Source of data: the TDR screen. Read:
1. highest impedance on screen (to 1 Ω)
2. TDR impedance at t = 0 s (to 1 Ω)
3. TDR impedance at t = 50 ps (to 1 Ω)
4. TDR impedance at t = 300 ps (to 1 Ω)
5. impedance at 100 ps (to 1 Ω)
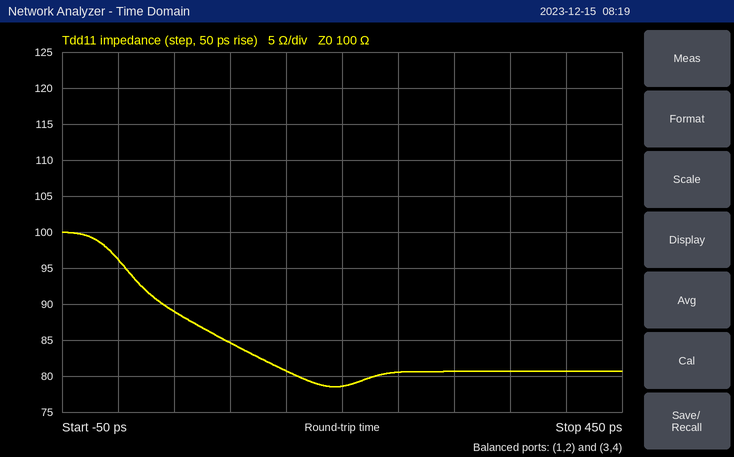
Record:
100 Ω
96 Ω
89 Ω
81 Ω
85 Ω
